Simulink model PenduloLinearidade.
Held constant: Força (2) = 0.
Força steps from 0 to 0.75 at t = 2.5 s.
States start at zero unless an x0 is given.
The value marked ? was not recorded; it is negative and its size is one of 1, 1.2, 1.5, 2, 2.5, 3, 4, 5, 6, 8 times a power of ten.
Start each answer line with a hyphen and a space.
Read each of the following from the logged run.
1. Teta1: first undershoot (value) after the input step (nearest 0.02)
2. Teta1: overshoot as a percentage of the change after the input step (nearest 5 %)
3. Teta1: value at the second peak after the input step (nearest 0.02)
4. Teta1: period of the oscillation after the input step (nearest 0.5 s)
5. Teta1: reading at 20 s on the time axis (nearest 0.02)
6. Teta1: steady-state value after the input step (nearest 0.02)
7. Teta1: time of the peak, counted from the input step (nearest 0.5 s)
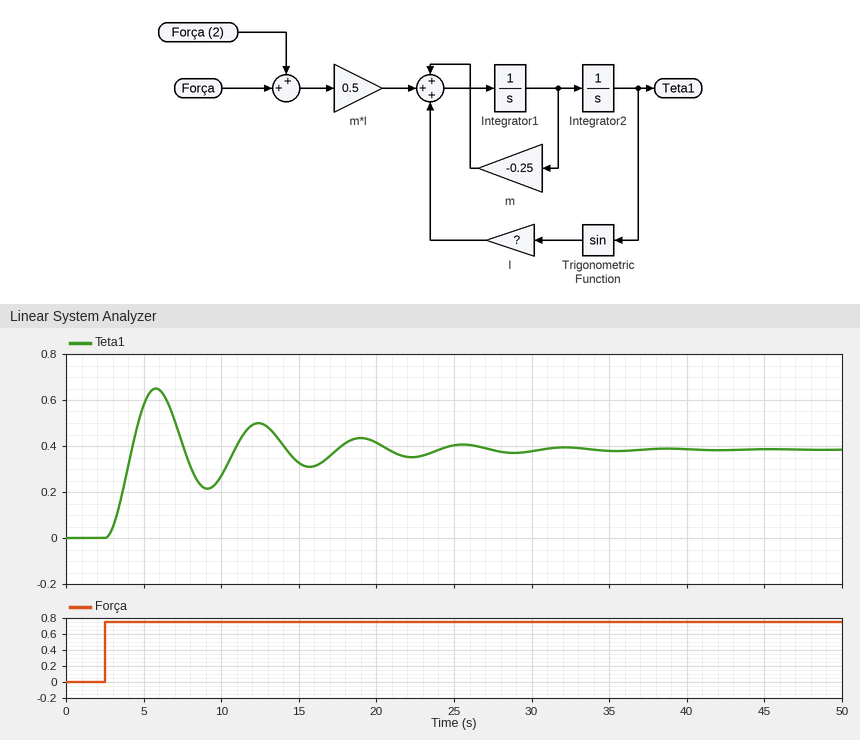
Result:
- 0.22
- 70 %
- 0.50
- 6.5 s
- 0.42
- 0.38
- 3.5 s
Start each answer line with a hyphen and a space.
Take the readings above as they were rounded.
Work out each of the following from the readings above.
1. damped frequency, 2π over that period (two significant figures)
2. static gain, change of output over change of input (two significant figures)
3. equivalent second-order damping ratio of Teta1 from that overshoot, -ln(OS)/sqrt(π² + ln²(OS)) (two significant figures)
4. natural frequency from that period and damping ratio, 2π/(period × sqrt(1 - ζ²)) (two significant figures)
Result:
- 0.97 rad/s
- 0.51
- 0.11
- 0.97 rad/s
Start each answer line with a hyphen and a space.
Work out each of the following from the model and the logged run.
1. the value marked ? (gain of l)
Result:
- -1
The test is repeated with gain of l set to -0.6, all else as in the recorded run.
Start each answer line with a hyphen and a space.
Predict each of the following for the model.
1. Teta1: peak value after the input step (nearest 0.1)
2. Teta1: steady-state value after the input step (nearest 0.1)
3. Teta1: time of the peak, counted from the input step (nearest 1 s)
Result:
- 1.1
- 0.7
- 5 s
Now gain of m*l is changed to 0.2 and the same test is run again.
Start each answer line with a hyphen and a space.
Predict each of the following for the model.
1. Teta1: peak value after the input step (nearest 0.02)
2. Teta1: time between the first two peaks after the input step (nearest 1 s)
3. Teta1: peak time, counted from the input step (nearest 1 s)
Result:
- 0.26
- 6 s
- 3 s
